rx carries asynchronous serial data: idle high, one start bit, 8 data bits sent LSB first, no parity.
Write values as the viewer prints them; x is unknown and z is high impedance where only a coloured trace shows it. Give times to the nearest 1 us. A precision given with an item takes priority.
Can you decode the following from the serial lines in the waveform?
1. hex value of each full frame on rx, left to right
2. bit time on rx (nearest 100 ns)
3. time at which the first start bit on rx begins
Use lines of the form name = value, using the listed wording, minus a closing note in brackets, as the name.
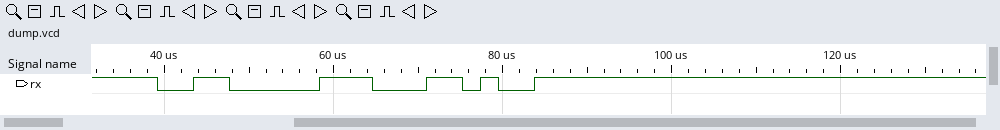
hex value of each full frame on rx, left to right = 06, 2C
bit time on rx = 2100 ns
time at which the first start bit on rx begins = 39 us
